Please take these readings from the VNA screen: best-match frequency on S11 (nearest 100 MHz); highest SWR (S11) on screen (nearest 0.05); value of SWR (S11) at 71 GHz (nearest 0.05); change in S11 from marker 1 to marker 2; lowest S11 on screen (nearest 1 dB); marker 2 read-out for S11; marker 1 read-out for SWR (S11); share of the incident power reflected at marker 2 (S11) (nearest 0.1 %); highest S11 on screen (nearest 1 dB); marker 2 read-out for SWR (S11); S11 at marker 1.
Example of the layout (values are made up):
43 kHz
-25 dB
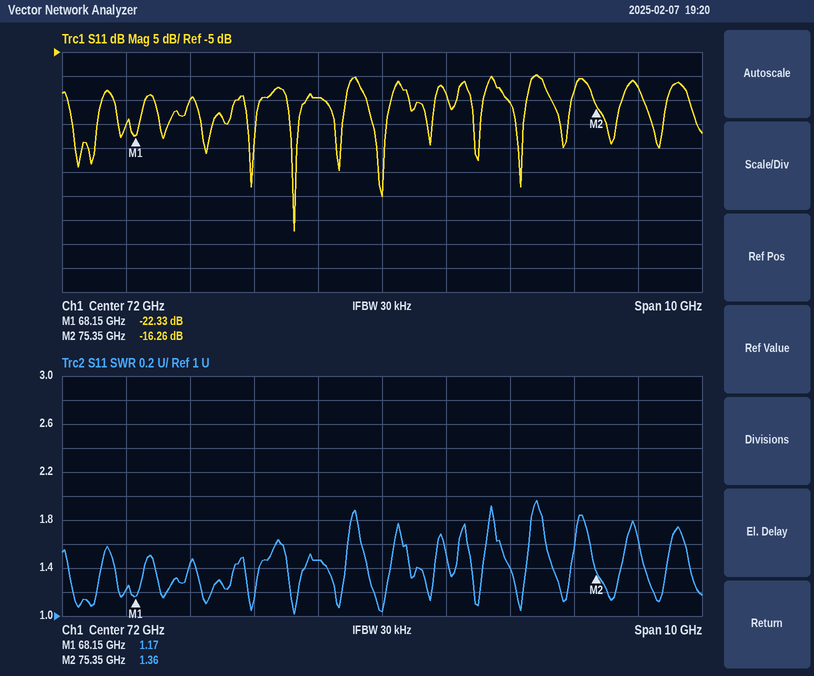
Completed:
70.6 GHz
1.95
1.45
6.07 dB
-42 dB
-16.26 dB
1.17
2.4 %
-10 dB
1.36
-22.33 dB
